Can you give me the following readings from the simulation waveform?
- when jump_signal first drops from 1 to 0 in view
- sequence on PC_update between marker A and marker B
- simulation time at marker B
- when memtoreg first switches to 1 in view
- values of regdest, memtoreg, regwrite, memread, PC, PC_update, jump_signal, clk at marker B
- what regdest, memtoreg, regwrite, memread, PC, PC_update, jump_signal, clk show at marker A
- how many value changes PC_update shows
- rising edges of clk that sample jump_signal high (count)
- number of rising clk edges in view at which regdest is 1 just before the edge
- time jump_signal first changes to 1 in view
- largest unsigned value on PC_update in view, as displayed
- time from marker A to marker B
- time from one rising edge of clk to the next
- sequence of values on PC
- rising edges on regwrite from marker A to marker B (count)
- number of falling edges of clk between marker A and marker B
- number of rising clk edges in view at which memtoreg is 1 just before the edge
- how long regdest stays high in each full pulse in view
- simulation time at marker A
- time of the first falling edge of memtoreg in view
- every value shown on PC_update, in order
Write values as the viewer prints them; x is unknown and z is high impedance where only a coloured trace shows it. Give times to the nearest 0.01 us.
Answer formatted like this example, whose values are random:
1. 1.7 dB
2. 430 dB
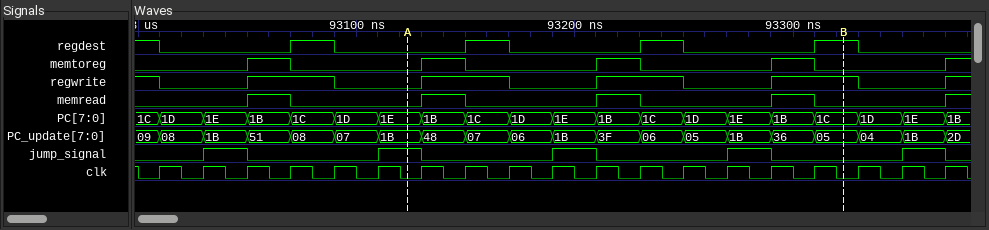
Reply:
1. 93.05 us
2. 1B, 48, 07, 06, 1B, 3F, 06, 05, 1B, 36, 05
3. 93.32 us
4. 93.05 us
5. regdest=1, memtoreg=0, regwrite=1, memread=0, PC=1C, PC_update=05, jump_signal=0, clk=0
6. regdest=0, memtoreg=0, regwrite=0, memread=0, PC=1E, PC_update=1B, jump_signal=1, clk=0
7. 19
8. 5
9. 5
10. 93.03 us
11. 51
12. 0.2 us
13. 0.02 us
14. 1C, 1D, 1E, 1B, 1C, 1D, 1E, 1B, 1C, 1D, 1E, 1B, 1C, 1D, 1E, 1B, 1C, 1D, 1E, 1B
15. 3
16. 10
17. 4
18. 0.02 us, 0.02 us, 0.02 us, 0.02 us
19. 93.12 us
20. 93.07 us
21. 09, 08, 1B, 51, 08, 07, 1B, 48, 07, 06, 1B, 3F, 06, 05, 1B, 36, 05, 04, 1B, 2D
